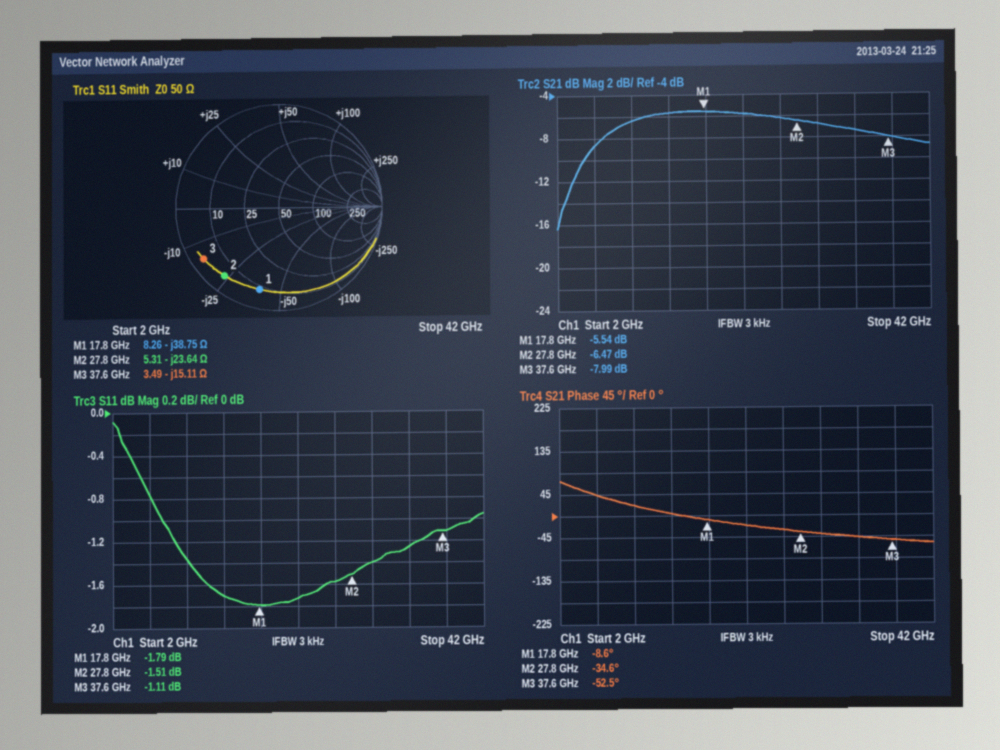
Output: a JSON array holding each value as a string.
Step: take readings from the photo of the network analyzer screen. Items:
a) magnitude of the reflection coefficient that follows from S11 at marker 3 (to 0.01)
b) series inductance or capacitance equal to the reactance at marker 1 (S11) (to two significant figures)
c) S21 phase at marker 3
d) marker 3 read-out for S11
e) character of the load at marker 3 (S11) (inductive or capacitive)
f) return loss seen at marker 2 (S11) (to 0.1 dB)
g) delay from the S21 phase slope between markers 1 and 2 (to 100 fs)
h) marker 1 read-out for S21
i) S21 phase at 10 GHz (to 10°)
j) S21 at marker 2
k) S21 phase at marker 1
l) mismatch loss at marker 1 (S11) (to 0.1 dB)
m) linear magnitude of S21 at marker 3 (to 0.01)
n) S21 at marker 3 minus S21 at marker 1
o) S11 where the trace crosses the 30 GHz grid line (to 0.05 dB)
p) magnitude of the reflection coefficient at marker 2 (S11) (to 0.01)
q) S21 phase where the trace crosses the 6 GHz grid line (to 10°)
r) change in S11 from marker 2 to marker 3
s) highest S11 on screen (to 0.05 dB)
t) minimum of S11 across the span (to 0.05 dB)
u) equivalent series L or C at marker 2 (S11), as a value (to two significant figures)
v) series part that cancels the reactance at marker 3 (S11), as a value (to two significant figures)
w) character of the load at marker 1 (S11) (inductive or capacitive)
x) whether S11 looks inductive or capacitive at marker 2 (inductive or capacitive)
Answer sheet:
["0.88", "230 fF", "-52.5°", "-1.11 dB", "capacitive", "1.5 dB", "7.2 ps", "-5.54 dB", "20°", "-6.47 dB", "-8.6°", "4.7 dB", "0.40", "-2.45 dB", "-1.40 dB", "0.84", "40°", "0.40 dB", "-0.10 dB", "-1.80 dB", "240 fF", "64 pH", "capacitive", "capacitive"]
